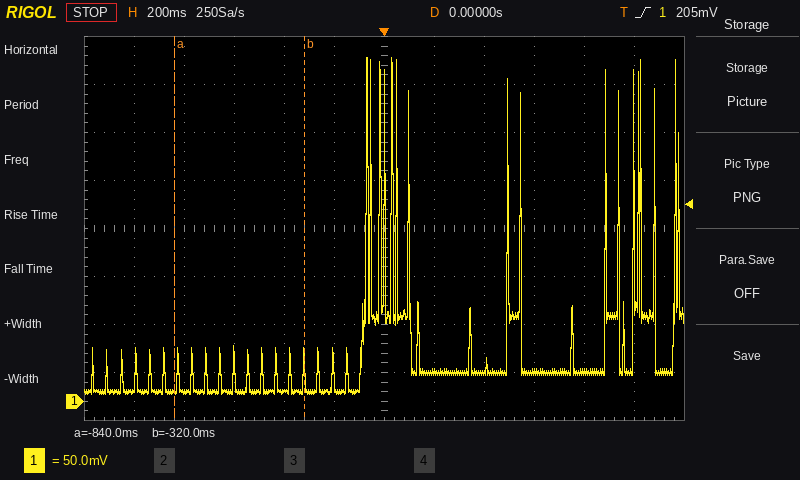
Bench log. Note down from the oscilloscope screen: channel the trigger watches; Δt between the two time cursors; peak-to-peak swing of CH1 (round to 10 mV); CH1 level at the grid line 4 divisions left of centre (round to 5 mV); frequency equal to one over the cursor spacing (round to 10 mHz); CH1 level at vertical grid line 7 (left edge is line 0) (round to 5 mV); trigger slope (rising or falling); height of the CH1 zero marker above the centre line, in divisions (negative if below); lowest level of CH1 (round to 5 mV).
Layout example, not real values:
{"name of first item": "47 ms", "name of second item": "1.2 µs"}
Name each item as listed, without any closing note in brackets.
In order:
{"channel the trigger watches": "CH1", "Δt between the two time cursors": "520 ms", "peak-to-peak swing of CH1": "350 mV", "CH1 level at the grid line 4 divisions left of centre": "10 mV", "frequency equal to one over the cursor spacing": "1.92 Hz", "CH1 level at vertical grid line 7 (left edge is line 0)": "30 mV", "trigger slope": "rising", "height of the CH1 zero marker above the centre line, in divisions": "-3.6 div", "lowest level of CH1": "10 mV"}
